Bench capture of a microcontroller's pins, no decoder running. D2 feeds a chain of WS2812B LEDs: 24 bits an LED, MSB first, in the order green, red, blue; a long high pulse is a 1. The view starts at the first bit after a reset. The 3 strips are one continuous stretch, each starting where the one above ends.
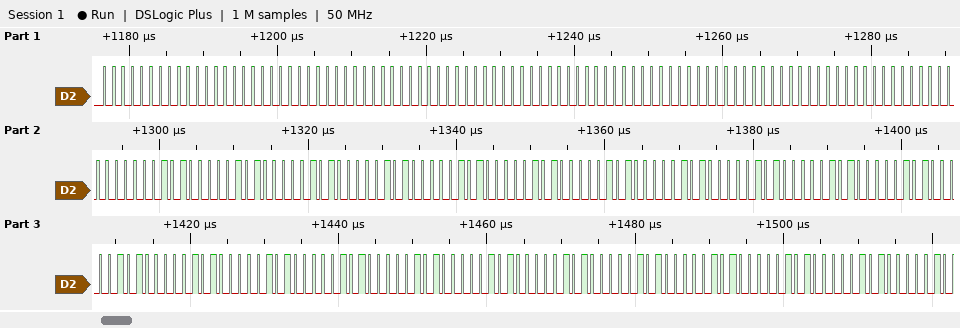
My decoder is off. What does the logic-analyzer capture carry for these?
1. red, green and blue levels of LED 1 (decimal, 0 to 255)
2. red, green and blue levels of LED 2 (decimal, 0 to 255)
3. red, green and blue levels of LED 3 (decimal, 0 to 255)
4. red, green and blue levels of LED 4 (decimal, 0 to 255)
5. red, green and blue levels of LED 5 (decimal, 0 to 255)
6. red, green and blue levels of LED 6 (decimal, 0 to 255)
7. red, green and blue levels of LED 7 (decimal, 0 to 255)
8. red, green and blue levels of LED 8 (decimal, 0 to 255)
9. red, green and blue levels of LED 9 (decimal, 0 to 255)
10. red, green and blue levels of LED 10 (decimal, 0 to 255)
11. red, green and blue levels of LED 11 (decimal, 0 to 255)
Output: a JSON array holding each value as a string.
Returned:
["0, 0, 0", "0, 0, 0", "0, 0, 0", "0, 0, 0", "20, 20, 20", "20, 20, 20", "20, 20, 20", "20, 20, 20", "20, 20, 20", "20, 20, 20", "20, 20, 20"]
